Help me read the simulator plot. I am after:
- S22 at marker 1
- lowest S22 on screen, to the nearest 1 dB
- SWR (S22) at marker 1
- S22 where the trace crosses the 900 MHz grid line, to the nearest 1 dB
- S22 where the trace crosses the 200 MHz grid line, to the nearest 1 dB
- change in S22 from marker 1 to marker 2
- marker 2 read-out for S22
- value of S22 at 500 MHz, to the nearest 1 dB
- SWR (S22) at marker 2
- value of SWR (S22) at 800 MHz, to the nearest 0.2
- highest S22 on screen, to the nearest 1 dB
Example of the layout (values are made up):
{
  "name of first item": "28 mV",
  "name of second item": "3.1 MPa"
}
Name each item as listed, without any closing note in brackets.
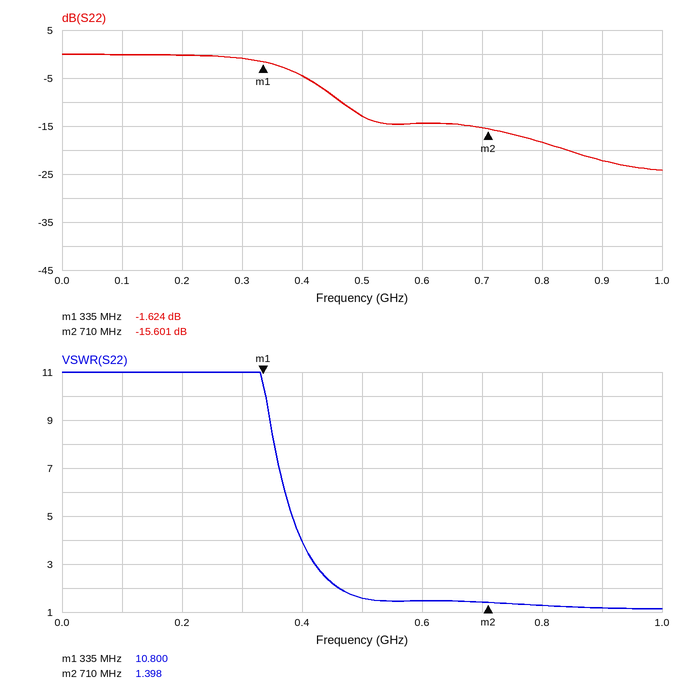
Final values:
{
  "S22 at marker 1": "-1.624 dB",
  "lowest S22 on screen, to the nearest 1 dB": "-24 dB",
  "SWR (S22) at marker 1": "10.800",
  "S22 where the trace crosses the 900 MHz grid line, to the nearest 1 dB": "-22 dB",
  "S22 where the trace crosses the 200 MHz grid line, to the nearest 1 dB": "0 dB",
  "change in S22 from marker 1 to marker 2": "-13.977 dB",
  "marker 2 read-out for S22": "-15.601 dB",
  "value of S22 at 500 MHz, to the nearest 1 dB": "-13 dB",
  "SWR (S22) at marker 2": "1.398",
  "value of SWR (S22) at 800 MHz, to the nearest 0.2": "1.2",
  "highest S22 on screen, to the nearest 1 dB": "0 dB"
}
